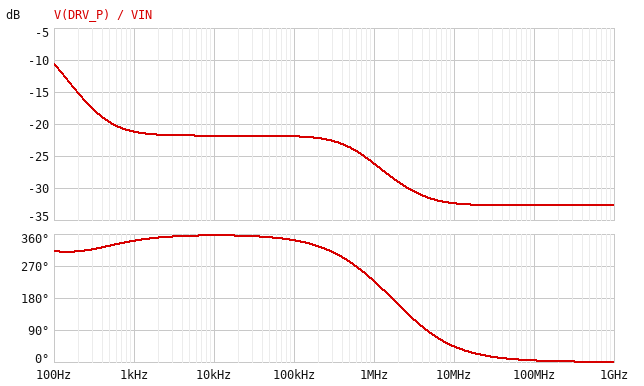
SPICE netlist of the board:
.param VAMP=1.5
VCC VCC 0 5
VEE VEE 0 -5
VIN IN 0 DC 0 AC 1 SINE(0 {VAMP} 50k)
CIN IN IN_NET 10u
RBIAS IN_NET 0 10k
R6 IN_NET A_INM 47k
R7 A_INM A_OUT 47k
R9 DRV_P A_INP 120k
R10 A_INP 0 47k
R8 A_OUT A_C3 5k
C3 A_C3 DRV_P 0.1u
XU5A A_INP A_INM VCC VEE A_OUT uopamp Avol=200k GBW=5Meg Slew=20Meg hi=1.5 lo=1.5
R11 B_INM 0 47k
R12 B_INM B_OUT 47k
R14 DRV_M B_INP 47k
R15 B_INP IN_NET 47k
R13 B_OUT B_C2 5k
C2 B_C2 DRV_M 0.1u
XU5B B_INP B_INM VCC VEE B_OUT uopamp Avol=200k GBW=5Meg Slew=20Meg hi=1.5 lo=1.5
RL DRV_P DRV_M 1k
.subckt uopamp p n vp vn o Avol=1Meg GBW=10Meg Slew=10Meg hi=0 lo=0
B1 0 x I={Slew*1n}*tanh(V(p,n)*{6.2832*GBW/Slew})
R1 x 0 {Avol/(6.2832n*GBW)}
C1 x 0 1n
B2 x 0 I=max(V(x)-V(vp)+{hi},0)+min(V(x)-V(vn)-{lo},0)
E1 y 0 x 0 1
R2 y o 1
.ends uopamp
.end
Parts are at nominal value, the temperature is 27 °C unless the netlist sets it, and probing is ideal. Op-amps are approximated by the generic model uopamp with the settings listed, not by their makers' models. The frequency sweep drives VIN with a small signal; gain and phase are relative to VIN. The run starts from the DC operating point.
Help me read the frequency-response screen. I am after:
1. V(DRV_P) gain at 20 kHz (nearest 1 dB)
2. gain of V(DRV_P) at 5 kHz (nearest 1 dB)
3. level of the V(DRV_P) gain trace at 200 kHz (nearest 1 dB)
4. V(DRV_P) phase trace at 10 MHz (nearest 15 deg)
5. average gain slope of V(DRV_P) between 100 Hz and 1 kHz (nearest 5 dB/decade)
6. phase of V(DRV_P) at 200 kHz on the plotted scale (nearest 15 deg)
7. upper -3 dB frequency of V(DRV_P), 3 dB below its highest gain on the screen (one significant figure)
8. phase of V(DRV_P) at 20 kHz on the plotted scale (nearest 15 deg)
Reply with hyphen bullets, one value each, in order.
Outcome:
- -22 dB
- -22 dB
- -22 dB
- 45 deg
- -10 dB/decade
- 330 deg
- 200 Hz
- 360 deg
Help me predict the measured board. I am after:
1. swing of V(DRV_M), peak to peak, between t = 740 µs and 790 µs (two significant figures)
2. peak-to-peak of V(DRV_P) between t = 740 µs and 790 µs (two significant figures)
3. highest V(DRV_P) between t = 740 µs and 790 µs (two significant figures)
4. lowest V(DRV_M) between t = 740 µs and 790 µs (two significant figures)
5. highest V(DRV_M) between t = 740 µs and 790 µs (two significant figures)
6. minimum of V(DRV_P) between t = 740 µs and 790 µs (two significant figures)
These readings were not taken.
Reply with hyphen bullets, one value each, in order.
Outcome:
- 860 mV
- 240 mV
- 120 mV
- -430 mV
- 430 mV
- -120 mV
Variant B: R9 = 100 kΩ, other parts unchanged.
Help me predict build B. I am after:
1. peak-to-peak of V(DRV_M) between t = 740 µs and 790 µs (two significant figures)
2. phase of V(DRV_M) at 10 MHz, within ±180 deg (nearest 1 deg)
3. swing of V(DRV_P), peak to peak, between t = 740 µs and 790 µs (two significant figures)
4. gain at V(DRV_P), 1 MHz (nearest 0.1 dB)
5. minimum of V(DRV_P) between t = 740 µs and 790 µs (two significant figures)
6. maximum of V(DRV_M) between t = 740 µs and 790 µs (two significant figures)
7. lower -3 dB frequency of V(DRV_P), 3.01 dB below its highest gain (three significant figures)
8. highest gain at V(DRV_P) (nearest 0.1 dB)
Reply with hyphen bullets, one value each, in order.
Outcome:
- 900 mV
- -40 deg
- 280 mV
- -25.8 dB
- -140 mV
- 450 mV
- 1.82 Hz
- -4.6 dB
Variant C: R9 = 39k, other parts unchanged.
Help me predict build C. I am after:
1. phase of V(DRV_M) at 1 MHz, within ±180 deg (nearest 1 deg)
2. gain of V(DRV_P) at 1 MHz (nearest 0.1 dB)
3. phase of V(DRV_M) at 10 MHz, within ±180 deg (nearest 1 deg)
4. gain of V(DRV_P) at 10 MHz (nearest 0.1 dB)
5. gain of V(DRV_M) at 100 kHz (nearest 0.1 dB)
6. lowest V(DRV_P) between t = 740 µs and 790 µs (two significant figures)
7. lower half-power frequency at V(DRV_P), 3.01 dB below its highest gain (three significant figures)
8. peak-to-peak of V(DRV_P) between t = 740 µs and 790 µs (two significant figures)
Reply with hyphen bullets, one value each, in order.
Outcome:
- -38 deg
- -24.7 dB
- -40 deg
- -32.5 dB
- -5.2 dB
- -1.4 V
- 1.76 kHz
- 2.8 V
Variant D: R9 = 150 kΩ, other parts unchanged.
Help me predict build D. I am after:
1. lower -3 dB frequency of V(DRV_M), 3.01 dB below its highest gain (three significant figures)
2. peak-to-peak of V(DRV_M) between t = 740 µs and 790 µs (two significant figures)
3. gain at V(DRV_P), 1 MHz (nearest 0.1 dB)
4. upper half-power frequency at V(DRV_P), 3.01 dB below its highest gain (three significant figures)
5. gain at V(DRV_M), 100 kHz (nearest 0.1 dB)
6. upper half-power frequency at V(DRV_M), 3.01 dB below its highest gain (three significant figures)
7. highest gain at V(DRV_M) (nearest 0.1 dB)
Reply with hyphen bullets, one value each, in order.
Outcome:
- 1.76 Hz
- 830 mV
- -26.6 dB
- 45.7 Hz
- -11.2 dB
- 43.5 Hz
- -3.8 dB
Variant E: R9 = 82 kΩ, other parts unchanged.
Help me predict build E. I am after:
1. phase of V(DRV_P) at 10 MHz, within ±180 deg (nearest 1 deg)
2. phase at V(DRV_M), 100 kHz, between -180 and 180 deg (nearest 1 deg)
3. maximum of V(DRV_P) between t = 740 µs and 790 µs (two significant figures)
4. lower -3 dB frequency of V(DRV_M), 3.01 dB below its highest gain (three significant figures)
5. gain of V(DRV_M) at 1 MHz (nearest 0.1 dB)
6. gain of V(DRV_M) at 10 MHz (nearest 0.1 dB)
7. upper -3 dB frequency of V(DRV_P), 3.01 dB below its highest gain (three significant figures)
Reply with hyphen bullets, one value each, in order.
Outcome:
- 43 deg
- -9 deg
- 170 mV
- 1.84 Hz
- -15.5 dB
- -27.5 dB
- 87.9 Hz
